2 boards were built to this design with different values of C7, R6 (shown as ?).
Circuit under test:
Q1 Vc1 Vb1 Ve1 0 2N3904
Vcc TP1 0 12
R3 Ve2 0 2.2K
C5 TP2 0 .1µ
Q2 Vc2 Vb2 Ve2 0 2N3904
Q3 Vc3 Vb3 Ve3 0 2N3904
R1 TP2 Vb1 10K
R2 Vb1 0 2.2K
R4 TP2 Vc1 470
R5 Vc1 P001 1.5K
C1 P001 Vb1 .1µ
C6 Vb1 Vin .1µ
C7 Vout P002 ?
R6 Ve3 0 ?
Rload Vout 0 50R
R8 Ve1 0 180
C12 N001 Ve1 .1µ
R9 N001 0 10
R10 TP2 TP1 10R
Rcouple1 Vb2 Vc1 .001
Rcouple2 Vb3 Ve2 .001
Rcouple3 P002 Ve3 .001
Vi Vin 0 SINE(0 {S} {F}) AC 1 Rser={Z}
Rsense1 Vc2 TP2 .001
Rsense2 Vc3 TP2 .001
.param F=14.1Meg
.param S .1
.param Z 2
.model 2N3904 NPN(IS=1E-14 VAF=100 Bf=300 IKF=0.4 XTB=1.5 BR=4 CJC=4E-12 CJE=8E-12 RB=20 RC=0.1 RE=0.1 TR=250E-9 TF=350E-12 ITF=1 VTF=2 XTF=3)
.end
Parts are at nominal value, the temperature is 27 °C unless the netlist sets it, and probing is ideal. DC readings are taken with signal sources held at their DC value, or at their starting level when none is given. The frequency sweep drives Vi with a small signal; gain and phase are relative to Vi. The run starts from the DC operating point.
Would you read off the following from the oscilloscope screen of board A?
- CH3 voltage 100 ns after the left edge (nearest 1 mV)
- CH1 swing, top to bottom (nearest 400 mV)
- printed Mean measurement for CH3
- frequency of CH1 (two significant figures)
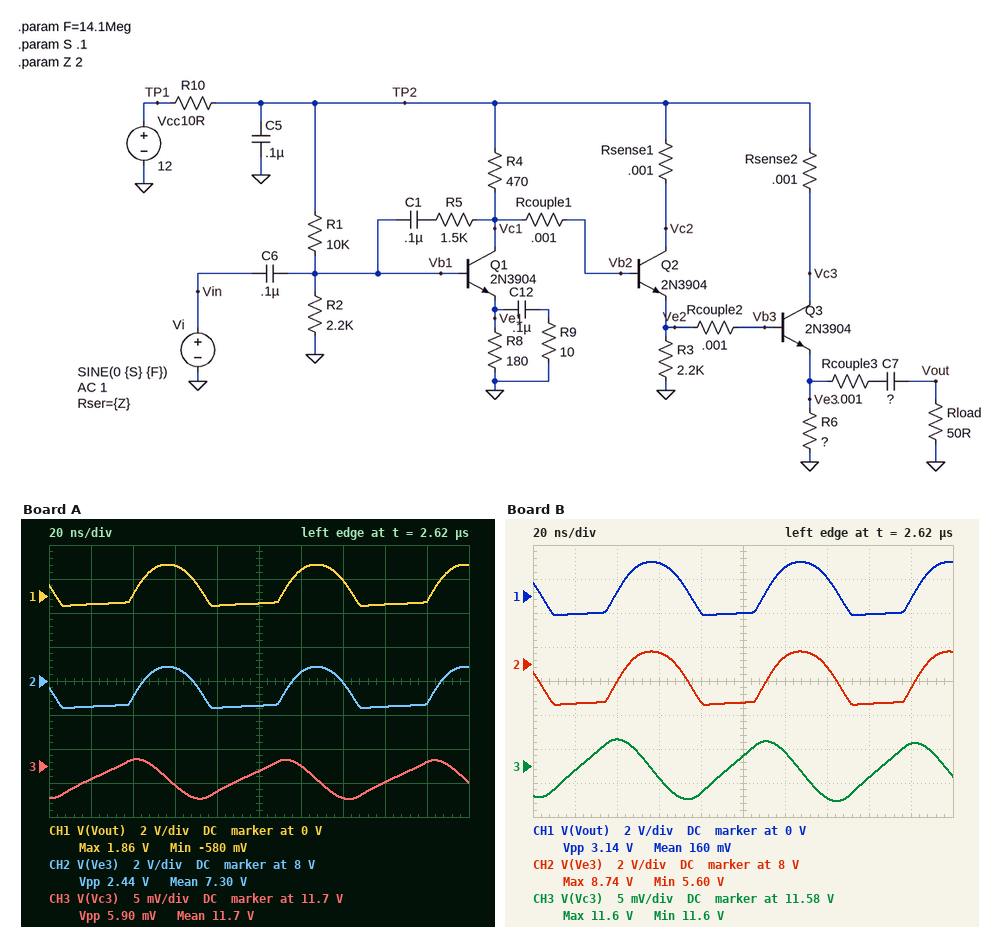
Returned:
11.699 V
2.4 V
11.7 V
14 MHz
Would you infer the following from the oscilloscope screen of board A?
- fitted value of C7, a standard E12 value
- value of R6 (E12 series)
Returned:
120 nF
680 Ω
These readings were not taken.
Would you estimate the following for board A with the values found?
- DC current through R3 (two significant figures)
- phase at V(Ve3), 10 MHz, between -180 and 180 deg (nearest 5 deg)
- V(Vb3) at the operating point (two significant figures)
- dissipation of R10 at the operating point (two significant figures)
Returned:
3.4 mA
165 deg
7.5 V
4.8 mW
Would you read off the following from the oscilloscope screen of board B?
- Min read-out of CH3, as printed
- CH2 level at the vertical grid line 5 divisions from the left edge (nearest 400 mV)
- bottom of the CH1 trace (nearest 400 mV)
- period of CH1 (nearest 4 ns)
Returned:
11.6 V
5.6 V
-1.2 V
72 ns
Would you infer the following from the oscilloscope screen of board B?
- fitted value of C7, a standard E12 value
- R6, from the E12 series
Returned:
270 nF
270 Ω
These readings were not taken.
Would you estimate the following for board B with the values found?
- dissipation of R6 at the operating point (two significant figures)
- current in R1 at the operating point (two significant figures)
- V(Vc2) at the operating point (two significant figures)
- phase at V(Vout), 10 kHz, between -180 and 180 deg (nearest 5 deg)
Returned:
170 mW
960 µA
12 V
-70 deg
